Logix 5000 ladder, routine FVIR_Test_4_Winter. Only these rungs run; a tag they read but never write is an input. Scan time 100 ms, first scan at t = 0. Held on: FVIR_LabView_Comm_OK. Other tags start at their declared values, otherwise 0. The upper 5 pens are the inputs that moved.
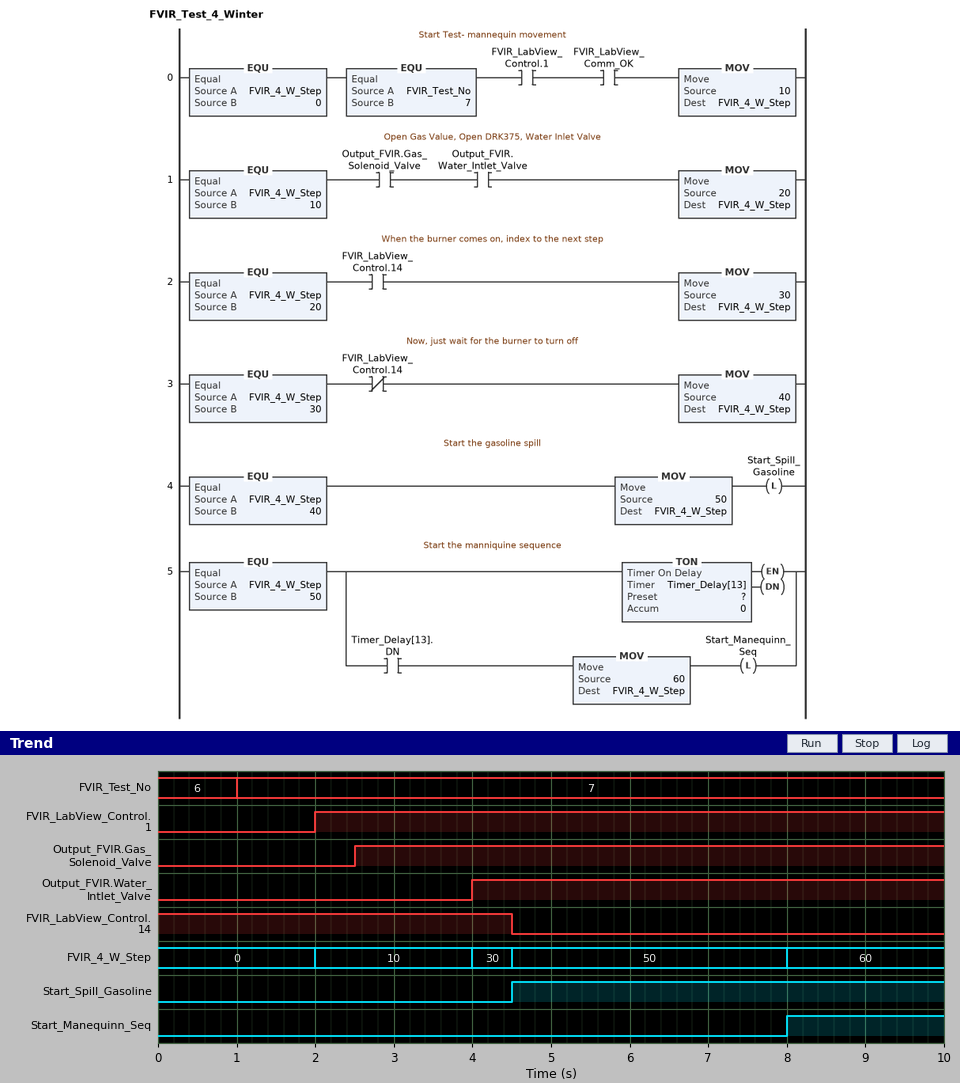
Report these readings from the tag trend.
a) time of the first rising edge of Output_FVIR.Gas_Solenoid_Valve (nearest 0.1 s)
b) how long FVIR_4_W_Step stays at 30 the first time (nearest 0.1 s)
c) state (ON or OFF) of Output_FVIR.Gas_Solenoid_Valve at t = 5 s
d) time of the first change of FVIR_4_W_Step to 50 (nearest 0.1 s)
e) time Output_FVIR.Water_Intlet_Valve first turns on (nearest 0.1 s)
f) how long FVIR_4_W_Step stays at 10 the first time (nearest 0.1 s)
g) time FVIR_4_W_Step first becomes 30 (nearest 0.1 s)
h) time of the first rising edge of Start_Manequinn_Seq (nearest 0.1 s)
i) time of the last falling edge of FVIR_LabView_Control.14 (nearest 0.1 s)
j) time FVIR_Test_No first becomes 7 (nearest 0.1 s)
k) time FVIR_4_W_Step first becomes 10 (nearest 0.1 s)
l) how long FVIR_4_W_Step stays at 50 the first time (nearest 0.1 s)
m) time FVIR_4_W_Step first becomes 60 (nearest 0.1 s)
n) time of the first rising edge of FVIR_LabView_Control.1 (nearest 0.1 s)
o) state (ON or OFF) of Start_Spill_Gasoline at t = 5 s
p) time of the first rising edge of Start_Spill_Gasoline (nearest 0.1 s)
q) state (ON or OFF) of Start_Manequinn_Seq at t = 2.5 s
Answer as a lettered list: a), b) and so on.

a) 2.5 s
b) 0.5 s
c) ON
d) 4.5 s
e) 4.0 s
f) 2.0 s
g) 4.0 s
h) 8.0 s
i) 4.5 s
j) 1.0 s
k) 2.0 s
l) 3.5 s
m) 8.0 s
n) 2.0 s
o) ON
p) 4.5 s
q) OFF
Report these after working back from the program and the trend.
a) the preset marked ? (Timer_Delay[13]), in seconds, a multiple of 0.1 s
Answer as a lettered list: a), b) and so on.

a) 3.5 s
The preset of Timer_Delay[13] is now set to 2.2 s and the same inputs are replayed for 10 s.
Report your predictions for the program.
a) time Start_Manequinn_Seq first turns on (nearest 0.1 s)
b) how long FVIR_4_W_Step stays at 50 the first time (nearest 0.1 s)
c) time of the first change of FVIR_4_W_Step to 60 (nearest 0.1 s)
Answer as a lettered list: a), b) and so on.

a) 6.7 s
b) 2.2 s
c) 6.7 s
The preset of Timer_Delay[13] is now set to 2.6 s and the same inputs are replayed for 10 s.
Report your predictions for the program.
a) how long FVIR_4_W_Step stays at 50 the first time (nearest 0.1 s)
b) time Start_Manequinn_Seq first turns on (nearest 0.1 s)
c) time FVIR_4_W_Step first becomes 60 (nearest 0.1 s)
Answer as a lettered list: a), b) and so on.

a) 2.6 s
b) 7.1 s
c) 7.1 s
